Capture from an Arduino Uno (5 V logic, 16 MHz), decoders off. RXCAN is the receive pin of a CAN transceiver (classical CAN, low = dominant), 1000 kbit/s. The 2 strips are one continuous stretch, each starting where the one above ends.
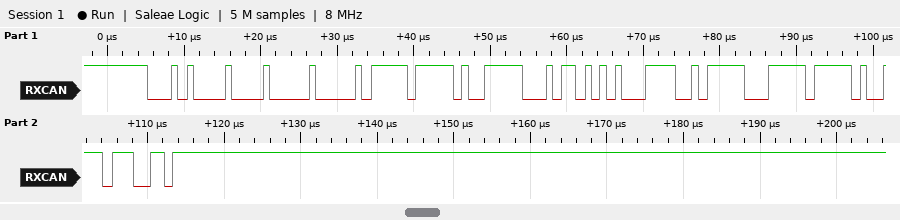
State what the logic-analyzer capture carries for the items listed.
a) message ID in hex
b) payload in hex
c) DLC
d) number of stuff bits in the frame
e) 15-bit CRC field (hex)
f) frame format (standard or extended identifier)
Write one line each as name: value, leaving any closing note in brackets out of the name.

message ID in hex: 0x142
payload in hex: 00 FF E7 CB 54 79 7C FF
DLC: 8
number of stuff bits in the frame: 8
15-bit CRC field: 0x73B9
frame format: standard
